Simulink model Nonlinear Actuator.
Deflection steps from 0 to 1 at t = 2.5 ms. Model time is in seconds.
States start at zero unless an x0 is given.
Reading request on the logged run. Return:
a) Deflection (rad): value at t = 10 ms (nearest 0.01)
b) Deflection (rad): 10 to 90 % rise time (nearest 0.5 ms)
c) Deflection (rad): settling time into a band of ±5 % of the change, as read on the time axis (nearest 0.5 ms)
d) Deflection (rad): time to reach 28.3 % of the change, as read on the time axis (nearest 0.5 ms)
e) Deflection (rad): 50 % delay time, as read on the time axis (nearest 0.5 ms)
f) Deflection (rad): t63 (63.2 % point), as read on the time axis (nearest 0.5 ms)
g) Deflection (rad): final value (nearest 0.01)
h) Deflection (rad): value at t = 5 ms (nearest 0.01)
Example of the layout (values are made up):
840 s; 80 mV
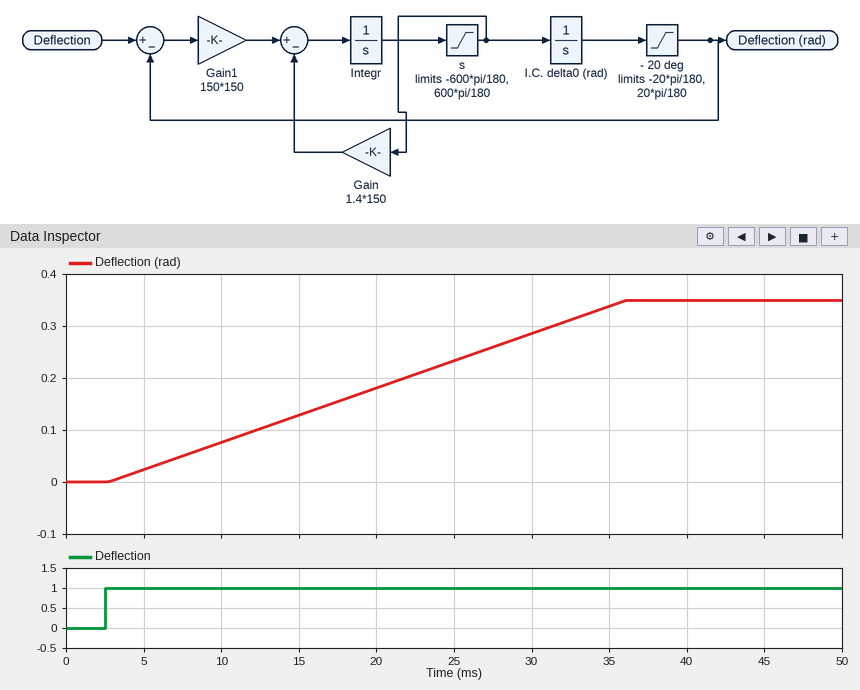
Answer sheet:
0.08; 26.5 ms; 34.5 ms; 12.0 ms; 19.5 ms; 24.0 ms; 0.35; 0.02
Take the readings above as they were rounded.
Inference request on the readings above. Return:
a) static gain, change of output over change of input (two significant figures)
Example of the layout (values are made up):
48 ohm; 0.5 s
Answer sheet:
0.35
